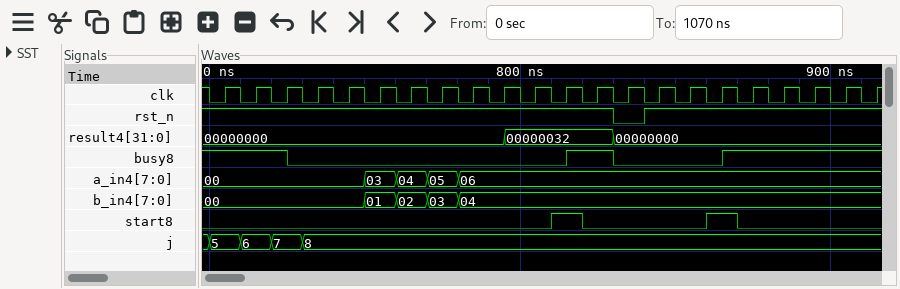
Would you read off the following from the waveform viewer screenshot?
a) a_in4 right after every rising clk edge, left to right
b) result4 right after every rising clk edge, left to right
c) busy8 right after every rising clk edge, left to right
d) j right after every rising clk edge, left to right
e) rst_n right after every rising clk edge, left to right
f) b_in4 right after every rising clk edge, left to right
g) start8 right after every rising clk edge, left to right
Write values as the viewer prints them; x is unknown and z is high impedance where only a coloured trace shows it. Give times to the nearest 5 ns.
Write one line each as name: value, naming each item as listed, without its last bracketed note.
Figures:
a_in4 right after every rising clk edge, left to right: 00, 00, 00, 00, 00, 03, 04, 05, 06, 06, 06, 06, 06, 06, 06, 06, 06, 06, 06, 06, 06, 06
result4 right after every rising clk edge, left to right: 00000000, 00000000, 00000000, 00000000, 00000000, 00000000, 00000000, 00000000, 00000000, 00000032, 00000032, 00000032, 00000032, 00000000, 00000000, 00000000, 00000000, 00000000, 00000000, 00000000, 00000000, 00000000
busy8 right after every rising clk edge, left to right: 1 1 0 0 0 0 0 0 0 0 0 1 1 0 0 0 1 1 1 1 1 1
j right after every rising clk edge, left to right: 5, 6, 7, 8, 8, 8, 8, 8, 8, 8, 8, 8, 8, 8, 8, 8, 8, 8, 8, 8, 8, 8
rst_n right after every rising clk edge, left to right: 1 1 1 1 1 1 1 1 1 1 1 1 1 0 1 1 1 1 1 1 1 1
b_in4 right after every rising clk edge, left to right: 00, 00, 00, 00, 00, 01, 02, 03, 04, 04, 04, 04, 04, 04, 04, 04, 04, 04, 04, 04, 04, 04
start8 right after every rising clk edge, left to right: 0 0 0 0 0 0 0 0 0 0 0 1 0 0 0 0 1 0 0 0 0 0
